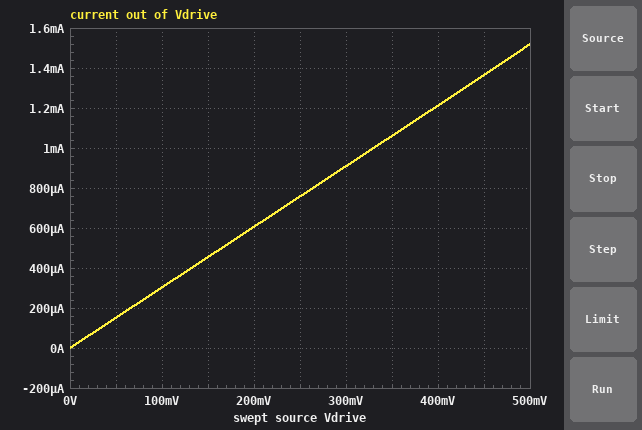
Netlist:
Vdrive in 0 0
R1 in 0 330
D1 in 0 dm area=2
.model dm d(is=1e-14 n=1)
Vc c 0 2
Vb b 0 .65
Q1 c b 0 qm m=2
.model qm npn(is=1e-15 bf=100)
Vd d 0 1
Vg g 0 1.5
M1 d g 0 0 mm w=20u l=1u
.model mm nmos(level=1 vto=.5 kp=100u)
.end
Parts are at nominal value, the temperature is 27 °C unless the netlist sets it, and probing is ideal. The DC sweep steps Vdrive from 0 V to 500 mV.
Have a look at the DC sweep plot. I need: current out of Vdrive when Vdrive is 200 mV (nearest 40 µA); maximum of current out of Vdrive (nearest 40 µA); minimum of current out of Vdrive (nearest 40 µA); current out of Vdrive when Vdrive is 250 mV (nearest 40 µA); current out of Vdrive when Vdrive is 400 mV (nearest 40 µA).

600 µA
1.52 mA
0 A
760 µA
1.20 mA
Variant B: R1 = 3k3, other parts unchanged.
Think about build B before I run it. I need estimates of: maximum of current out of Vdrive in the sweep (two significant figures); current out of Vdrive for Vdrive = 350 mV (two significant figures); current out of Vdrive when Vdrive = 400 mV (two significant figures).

160 µA
110 µA
120 µA
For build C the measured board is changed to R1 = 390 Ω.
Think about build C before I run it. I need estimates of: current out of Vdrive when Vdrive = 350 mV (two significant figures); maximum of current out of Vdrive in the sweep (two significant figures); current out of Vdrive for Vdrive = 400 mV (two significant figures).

900 µA
1.3 mA
1.0 mA
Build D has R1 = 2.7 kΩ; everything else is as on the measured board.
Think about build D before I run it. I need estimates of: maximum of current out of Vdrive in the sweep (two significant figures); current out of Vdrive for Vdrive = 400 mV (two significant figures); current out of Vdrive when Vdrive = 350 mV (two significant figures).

190 µA
150 µA
130 µA
